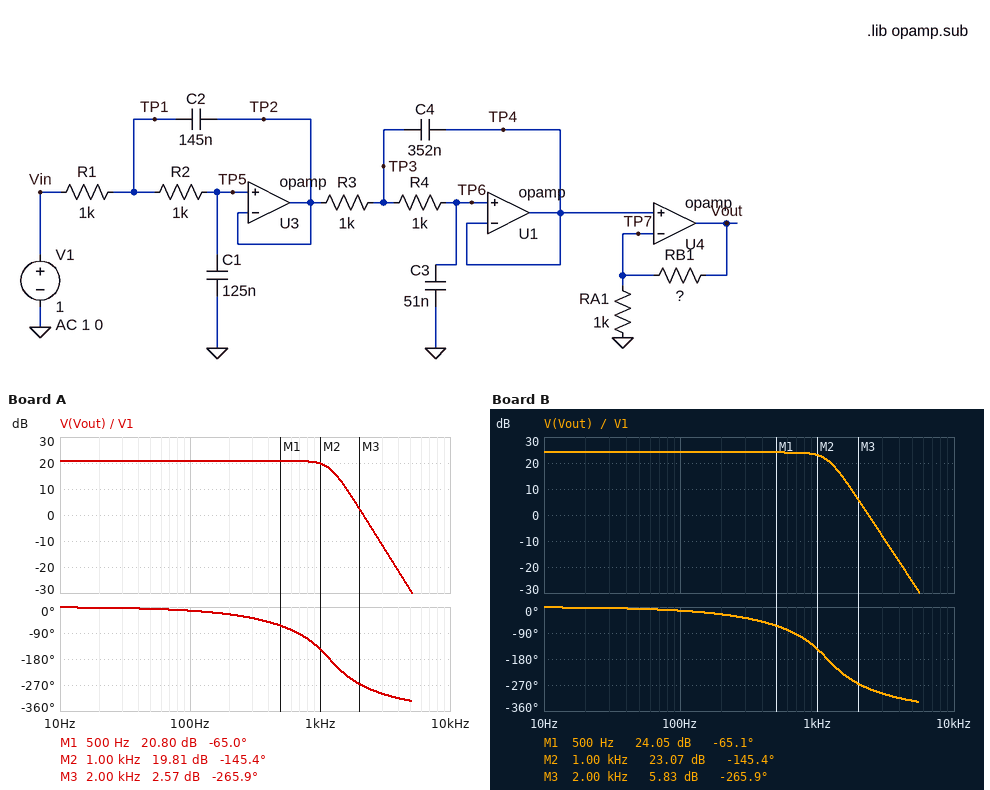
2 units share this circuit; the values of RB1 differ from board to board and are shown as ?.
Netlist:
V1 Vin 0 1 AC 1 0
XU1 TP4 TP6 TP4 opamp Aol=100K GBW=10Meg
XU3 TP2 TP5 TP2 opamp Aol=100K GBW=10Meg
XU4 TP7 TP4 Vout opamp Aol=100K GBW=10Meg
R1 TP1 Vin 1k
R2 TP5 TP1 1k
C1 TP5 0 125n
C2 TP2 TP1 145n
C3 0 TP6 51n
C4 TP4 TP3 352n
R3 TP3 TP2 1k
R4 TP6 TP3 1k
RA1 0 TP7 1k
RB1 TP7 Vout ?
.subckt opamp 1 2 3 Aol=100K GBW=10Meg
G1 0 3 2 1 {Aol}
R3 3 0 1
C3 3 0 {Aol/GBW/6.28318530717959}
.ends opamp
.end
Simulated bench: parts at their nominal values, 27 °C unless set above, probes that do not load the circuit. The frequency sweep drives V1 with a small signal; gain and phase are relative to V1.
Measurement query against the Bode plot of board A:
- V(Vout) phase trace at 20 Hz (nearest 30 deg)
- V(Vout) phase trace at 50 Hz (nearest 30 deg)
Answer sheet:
0 deg
0 deg
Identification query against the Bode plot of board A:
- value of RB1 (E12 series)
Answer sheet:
10 kΩ
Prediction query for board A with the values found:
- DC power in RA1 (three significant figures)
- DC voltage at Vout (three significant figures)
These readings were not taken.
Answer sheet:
1.00 mW
11.0 V
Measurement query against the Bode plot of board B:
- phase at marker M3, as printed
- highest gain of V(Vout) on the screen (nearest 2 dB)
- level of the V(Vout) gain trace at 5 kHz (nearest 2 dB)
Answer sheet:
-265.9 deg
24 dB
-26 dB
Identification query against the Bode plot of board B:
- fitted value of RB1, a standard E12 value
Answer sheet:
15 kΩ
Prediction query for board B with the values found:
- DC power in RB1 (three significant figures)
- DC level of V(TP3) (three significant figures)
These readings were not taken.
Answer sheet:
15.0 mW
1.00 V
